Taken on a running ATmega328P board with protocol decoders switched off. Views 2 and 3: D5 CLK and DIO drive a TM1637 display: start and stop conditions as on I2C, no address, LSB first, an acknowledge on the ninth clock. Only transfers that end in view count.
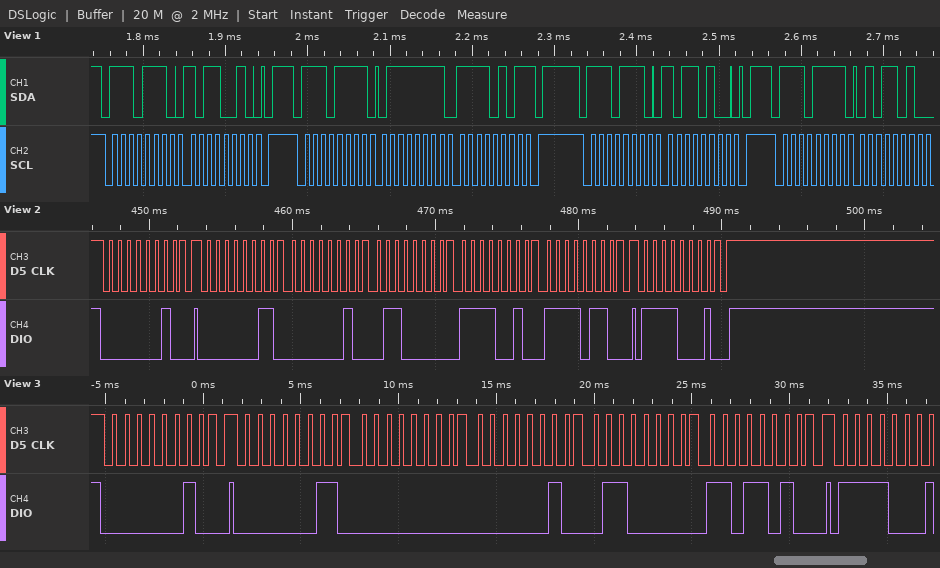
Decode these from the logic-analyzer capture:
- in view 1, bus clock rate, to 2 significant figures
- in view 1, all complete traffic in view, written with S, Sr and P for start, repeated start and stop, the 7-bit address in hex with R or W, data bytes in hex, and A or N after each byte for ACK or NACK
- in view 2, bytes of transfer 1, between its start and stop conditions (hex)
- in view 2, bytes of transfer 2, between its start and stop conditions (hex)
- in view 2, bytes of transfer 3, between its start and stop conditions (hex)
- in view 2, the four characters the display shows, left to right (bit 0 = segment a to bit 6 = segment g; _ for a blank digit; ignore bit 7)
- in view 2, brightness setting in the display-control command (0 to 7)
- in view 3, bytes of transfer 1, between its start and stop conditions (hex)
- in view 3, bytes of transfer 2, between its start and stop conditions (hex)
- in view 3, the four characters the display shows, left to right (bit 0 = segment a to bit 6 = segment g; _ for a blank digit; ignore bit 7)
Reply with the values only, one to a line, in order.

100 kHz
S 77W A B2 A P S 77R A 7F A F5 N P S 77W A B4 A P S 77R A 5A A
40
C0 40 06 4F 6F
8F
-139
7
40
C0 00 40 06 5B
_-12
